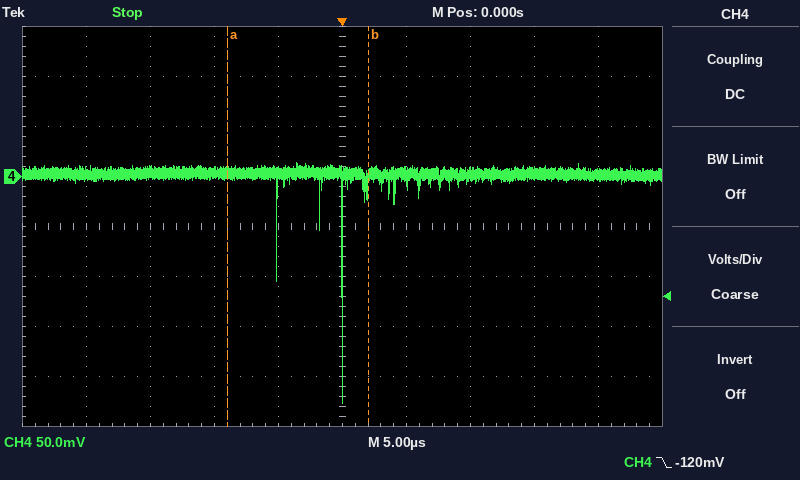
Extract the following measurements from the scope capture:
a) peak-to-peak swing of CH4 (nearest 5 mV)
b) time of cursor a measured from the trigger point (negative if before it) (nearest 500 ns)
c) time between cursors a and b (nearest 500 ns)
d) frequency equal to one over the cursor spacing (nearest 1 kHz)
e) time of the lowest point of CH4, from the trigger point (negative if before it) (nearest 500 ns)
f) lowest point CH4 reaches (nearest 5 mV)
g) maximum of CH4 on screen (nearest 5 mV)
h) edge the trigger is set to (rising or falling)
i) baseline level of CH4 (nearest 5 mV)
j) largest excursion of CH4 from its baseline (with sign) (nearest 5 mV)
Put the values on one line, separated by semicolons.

240 mV; -9.0 µs; 11.0 µs; 91 kHz; 0.0 µs; -225 mV; 15 mV; falling; 5 mV; -230 mV
